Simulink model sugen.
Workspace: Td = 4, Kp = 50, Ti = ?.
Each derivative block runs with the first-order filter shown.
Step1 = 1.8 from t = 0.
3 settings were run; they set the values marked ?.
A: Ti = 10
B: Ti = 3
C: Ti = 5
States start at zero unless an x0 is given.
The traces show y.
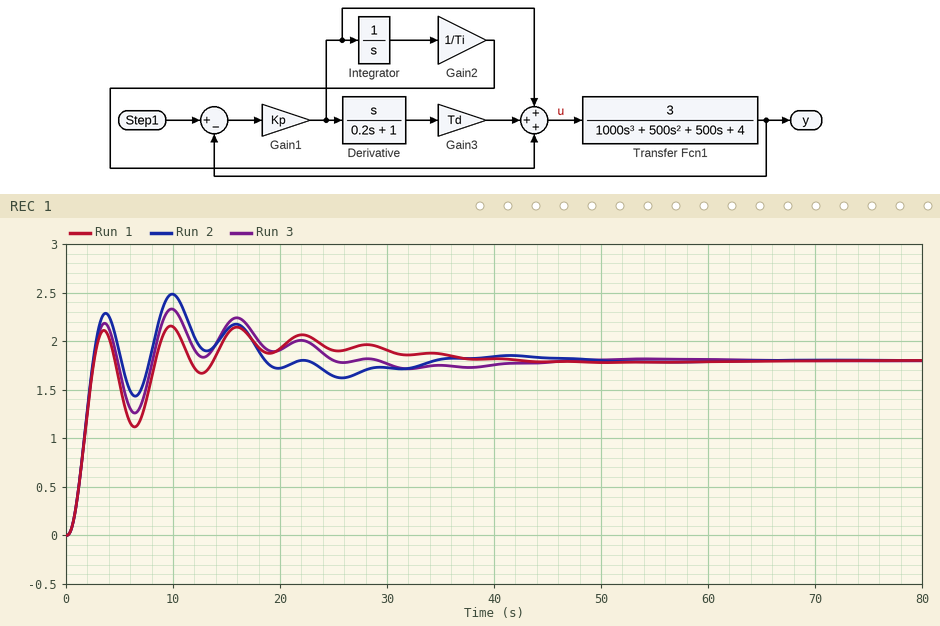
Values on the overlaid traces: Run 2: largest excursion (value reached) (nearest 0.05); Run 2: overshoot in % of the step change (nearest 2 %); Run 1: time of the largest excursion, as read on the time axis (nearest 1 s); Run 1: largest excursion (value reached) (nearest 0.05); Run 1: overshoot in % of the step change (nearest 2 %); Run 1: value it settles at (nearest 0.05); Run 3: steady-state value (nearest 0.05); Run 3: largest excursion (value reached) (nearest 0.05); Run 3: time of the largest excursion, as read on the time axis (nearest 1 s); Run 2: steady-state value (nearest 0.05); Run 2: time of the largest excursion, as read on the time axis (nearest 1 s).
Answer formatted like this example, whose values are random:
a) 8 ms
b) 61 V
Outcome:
a) 2.50
b) 38 %
c) 10 s
d) 2.15
e) 20 %
f) 1.80
g) 1.80
h) 2.35
i) 10 s
j) 1.80
k) 10 s
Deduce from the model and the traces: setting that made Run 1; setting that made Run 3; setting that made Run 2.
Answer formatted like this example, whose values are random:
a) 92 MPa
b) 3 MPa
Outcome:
a) A
b) C
c) B
